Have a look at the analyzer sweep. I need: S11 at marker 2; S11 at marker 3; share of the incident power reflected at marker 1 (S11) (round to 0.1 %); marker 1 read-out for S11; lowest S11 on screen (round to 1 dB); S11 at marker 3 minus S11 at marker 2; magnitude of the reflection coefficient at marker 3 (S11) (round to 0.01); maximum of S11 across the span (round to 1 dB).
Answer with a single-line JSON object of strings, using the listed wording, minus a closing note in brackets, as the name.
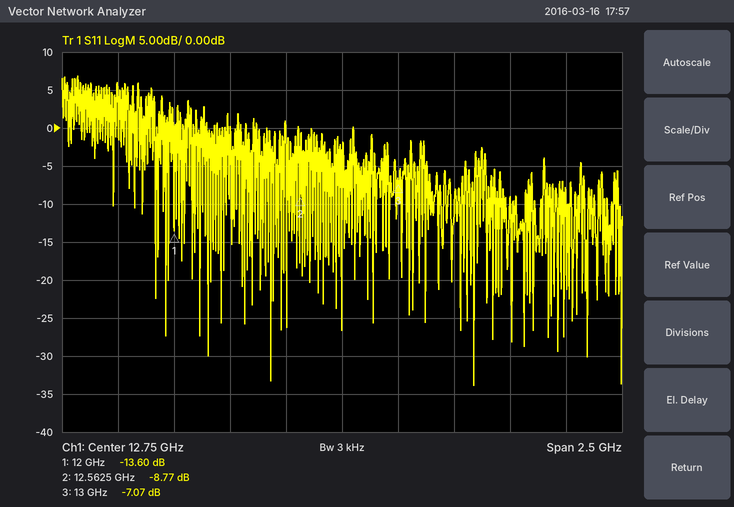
{"S11 at marker 2": "-8.77 dB", "S11 at marker 3": "-7.07 dB", "share of the incident power reflected at marker 1 (S11)": "4.4 %", "marker 1 read-out for S11": "-13.60 dB", "lowest S11 on screen": "-34 dB", "S11 at marker 3 minus S11 at marker 2": "1.70 dB", "magnitude of the reflection coefficient at marker 3 (S11)": "0.44", "maximum of S11 across the span": "7 dB"}
